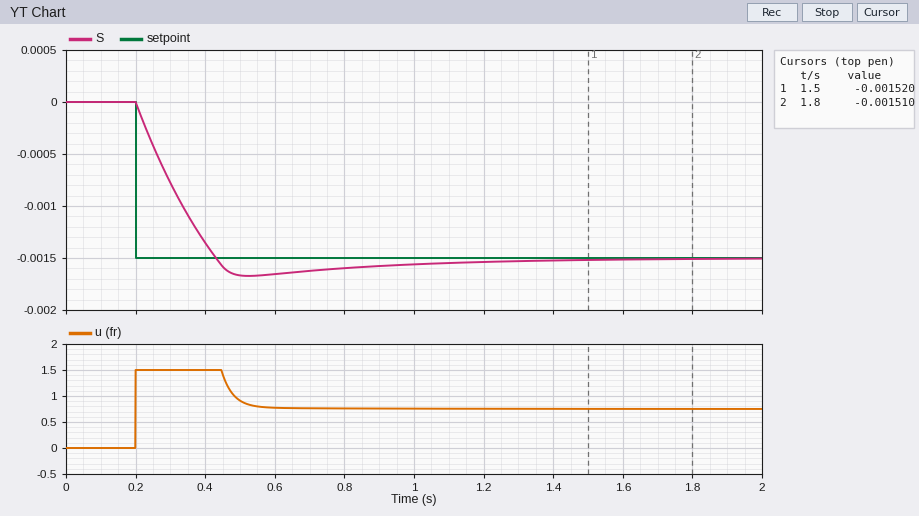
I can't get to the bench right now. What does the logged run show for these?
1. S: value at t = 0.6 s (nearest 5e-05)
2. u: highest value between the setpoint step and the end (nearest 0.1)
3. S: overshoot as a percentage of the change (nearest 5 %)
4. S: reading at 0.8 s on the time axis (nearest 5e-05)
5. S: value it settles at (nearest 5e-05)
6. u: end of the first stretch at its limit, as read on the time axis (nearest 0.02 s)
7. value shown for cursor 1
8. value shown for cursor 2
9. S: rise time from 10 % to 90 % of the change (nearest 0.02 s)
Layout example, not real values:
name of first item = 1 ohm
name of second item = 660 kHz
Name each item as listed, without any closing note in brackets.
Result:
S: value at t = 0.6 s = -0.00165
u: highest value between the setpoint step and the end = 1.5
S: overshoot as a percentage of the change = 10 %
S: reading at 0.8 s on the time axis = -0.00160
S: value it settles at = -0.00150
u: end of the first stretch at its limit, as read on the time axis = 0.44 s
value shown for cursor 1 = -0.001520
value shown for cursor 2 = -0.001510
S: rise time from 10 % to 90 % of the change = 0.18 s
